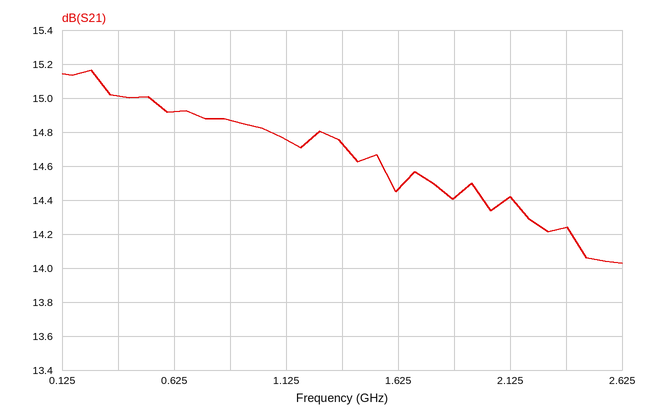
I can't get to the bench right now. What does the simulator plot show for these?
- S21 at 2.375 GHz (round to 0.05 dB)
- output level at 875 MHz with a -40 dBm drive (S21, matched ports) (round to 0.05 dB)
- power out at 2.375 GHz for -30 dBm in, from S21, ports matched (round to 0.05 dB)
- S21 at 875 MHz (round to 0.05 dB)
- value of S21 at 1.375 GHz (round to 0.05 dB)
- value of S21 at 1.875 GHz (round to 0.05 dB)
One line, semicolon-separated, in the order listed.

14.25 dB; -25.15 dBm; -15.75 dBm; 14.85 dB; 14.75 dB; 14.40 dB
